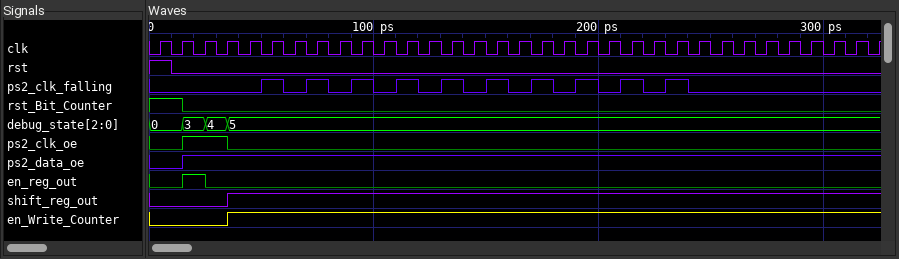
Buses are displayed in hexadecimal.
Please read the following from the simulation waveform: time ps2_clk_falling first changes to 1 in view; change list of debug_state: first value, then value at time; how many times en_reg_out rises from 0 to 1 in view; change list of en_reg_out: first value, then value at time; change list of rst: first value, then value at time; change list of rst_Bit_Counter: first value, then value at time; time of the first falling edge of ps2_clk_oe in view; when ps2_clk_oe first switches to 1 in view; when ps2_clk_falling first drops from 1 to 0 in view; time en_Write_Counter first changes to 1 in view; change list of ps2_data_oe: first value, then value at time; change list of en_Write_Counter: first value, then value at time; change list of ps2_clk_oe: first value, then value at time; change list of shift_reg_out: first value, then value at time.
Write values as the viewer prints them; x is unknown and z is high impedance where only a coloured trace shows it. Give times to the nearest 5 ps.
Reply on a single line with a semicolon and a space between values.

50 ps; 0, 3 at 15 ps, 4 at 25 ps, 5 at 35 ps; 1; 0, 1 at 15 ps, 0 at 25 ps; 1, 0 at 10 ps; 1, 0 at 15 ps; 35 ps; 15 ps; 60 ps; 35 ps; 0, 1 at 15 ps; 0, 1 at 35 ps; 0, 1 at 15 ps, 0 at 35 ps; 0, 1 at 35 ps
